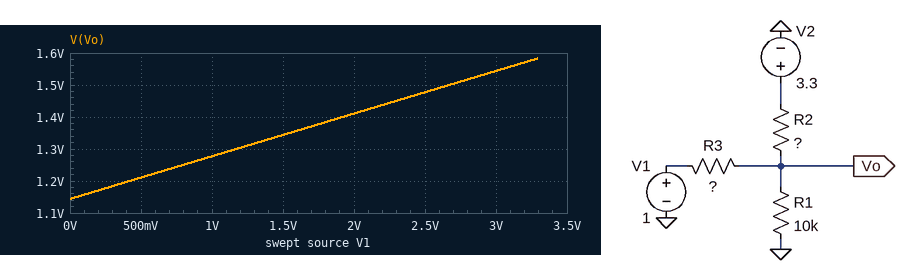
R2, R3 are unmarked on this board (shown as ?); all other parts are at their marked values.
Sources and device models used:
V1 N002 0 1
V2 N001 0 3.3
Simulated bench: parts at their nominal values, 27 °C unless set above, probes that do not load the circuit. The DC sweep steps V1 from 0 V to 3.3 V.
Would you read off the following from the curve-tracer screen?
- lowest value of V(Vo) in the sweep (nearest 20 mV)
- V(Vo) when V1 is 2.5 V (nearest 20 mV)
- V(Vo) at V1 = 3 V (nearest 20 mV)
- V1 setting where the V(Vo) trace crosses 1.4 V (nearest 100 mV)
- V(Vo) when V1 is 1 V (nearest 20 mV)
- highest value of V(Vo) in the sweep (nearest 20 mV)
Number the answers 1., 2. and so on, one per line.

1. 1.14 V
2. 1.48 V
3. 1.54 V
4. 1.9 V
5. 1.28 V
6. 1.58 V
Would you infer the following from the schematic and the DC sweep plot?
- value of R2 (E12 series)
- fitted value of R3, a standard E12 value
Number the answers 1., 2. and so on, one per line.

1. 15 kΩ
2. 39 kΩ
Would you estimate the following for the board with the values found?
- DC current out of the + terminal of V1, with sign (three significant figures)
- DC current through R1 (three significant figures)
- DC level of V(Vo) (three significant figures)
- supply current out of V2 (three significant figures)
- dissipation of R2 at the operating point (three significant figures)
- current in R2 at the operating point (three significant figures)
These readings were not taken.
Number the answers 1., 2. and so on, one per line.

1. -7.11 µA
2. 128 µA
3. 1.28 V
4. 135 µA
5. 273 µW
6. 135 µA
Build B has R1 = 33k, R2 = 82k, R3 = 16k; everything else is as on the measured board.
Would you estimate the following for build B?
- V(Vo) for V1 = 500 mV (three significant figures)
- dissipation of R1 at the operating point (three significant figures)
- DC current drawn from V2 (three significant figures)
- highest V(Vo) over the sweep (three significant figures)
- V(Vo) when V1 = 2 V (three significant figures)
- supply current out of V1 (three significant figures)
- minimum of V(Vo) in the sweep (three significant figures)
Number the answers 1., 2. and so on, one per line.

1. 681 mV
2. 29.0 µW
3. 28.3 µA
4. 2.35 V
5. 1.57 V
6. 1.34 µA
7. 383 mV
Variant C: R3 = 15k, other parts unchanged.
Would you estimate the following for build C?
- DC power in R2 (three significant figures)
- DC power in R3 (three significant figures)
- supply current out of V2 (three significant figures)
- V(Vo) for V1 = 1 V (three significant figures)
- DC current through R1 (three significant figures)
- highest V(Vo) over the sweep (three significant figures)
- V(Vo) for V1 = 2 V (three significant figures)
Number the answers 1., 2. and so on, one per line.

1. 286 µW
2. 3.48 µW
3. 138 µA
4. 1.23 V
5. 123 µA
6. 1.89 V
7. 1.51 V
